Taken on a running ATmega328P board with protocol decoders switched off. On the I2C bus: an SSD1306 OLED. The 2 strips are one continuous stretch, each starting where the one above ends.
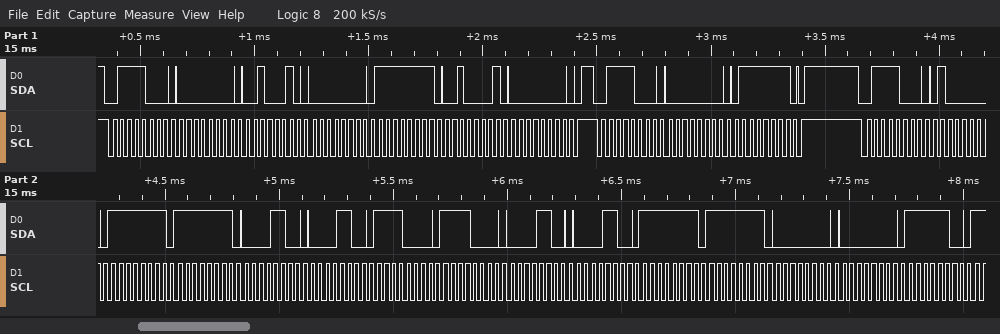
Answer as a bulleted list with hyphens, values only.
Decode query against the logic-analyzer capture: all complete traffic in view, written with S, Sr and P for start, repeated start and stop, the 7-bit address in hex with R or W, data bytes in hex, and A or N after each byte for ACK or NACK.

- S 3CW A 00 A 22 A 00 A FF A 21 A 00 A P S 3CW A 00 A 7F A P S 3CW A 40 A FF A FF A 0C A 0C A F0 A F0 A 0C A 0C A FF A FF A 00 A 00 A FC A
